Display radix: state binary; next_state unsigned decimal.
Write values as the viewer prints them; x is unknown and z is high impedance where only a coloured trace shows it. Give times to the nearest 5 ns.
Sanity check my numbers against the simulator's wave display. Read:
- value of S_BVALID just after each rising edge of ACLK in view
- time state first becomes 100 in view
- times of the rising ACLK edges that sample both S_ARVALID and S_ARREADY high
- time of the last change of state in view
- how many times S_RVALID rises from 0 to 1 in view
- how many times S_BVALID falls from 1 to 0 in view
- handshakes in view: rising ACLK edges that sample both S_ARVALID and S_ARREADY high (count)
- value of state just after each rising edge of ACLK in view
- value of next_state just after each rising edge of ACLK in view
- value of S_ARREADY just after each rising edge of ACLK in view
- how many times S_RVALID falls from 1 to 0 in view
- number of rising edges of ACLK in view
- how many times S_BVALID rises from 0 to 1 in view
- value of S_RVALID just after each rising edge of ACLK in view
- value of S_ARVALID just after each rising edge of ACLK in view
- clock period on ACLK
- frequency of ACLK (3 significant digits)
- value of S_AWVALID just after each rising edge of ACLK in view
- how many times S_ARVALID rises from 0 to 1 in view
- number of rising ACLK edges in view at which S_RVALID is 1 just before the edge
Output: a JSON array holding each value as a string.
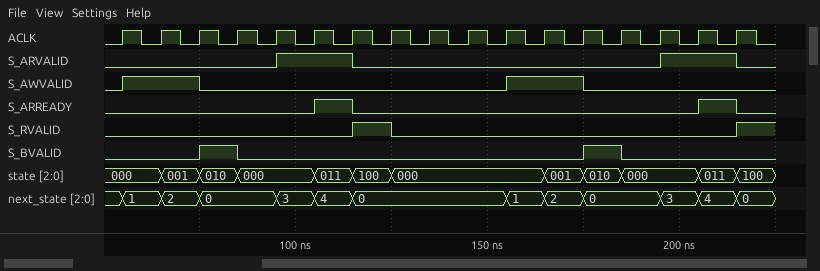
["0 0 1 0 0 0 0 0 0 0 0 0 1 0 0 0 0", "115 ns", "115 ns, 215 ns", "215 ns", "2", "2", "2", "000, 001, 010, 000, 000, 011, 100, 000, 000, 000, 000, 001, 010, 000, 000, 011, 100", "1, 2, 0, 0, 3, 4, 0, 0, 0, 0, 1, 2, 0, 0, 3, 4, 0", "0 0 0 0 0 1 0 0 0 0 0 0 0 0 0 1 0", "1", "17", "2", "0 0 0 0 0 0 1 0 0 0 0 0 0 0 0 0 1", "0 0 0 0 1 1 0 0 0 0 0 0 0 0 1 1 0", "10 ns", "100 MHz", "1 1 0 0 0 0 0 0 0 0 1 1 0 0 0 0 0", "2", "1"]
